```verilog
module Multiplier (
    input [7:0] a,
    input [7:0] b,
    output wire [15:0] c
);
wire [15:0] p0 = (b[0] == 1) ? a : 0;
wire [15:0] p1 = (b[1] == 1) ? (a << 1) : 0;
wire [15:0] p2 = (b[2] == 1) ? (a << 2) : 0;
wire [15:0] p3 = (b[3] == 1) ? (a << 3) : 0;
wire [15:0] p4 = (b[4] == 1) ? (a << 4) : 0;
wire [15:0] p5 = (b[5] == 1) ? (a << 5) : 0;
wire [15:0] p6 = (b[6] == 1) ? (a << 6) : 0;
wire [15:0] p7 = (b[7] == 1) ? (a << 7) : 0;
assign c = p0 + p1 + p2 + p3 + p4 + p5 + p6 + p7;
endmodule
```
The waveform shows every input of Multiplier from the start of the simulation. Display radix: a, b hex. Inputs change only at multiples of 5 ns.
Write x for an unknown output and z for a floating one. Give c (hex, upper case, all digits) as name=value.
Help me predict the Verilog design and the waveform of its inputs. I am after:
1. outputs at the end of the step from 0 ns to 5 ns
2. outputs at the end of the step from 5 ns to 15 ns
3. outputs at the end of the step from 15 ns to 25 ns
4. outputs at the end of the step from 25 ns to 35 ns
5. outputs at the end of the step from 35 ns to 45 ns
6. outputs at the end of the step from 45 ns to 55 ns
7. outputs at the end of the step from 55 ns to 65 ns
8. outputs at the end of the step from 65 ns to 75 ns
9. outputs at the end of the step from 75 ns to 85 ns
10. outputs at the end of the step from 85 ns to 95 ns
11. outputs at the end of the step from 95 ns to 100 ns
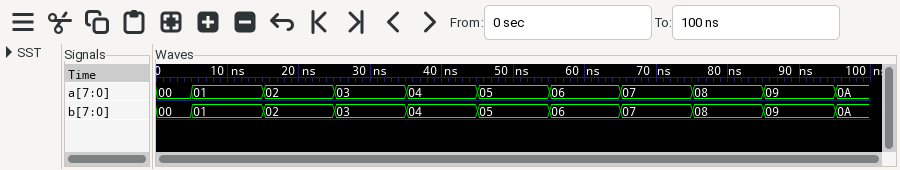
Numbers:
c=0000
c=0001
c=0004
c=0009
c=0010
c=0019
c=0024
c=0031
c=0040
c=0051
c=0064
